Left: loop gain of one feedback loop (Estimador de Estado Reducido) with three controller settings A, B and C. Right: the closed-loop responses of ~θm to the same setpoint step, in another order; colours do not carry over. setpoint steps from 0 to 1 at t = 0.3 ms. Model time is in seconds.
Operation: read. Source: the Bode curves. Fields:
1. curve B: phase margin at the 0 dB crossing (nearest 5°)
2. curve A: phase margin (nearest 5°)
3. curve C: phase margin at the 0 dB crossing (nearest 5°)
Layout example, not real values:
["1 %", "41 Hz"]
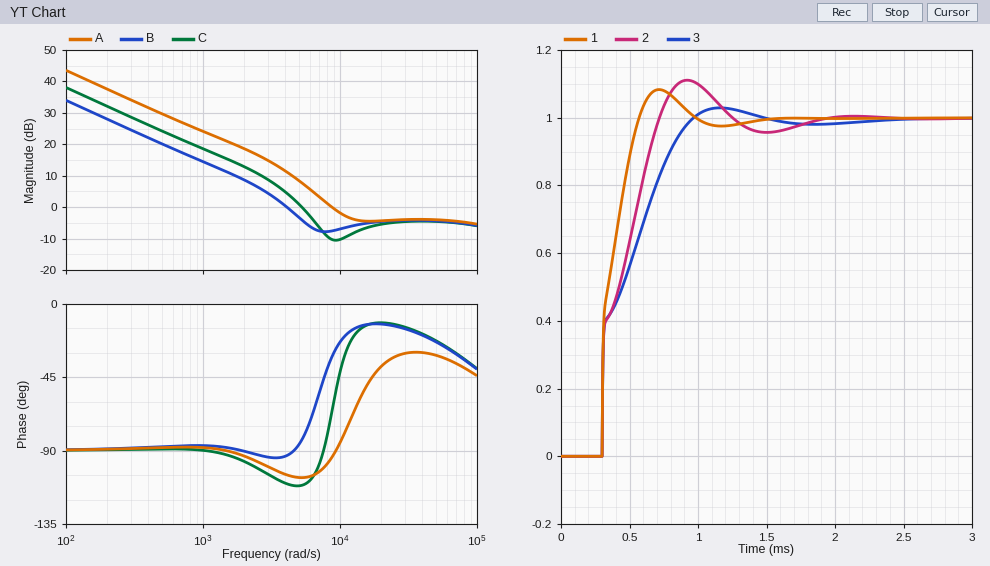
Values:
["85°", "85°", "70°"]
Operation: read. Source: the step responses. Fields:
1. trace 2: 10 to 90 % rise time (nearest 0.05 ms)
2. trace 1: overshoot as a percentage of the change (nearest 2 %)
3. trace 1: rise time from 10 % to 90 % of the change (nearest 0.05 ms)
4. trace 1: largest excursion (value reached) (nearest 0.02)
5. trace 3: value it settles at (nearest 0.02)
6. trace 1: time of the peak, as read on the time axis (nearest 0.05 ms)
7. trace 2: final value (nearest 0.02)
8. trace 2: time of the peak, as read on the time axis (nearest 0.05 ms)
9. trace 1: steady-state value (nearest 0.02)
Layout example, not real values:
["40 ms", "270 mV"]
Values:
["0.35 ms", "8 %", "0.20 ms", "1.08", "1.00", "0.70 ms", "1.00", "0.90 ms", "1.00"]
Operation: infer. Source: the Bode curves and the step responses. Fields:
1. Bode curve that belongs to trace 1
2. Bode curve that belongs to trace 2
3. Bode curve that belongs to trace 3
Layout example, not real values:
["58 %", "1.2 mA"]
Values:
["A", "C", "B"]
